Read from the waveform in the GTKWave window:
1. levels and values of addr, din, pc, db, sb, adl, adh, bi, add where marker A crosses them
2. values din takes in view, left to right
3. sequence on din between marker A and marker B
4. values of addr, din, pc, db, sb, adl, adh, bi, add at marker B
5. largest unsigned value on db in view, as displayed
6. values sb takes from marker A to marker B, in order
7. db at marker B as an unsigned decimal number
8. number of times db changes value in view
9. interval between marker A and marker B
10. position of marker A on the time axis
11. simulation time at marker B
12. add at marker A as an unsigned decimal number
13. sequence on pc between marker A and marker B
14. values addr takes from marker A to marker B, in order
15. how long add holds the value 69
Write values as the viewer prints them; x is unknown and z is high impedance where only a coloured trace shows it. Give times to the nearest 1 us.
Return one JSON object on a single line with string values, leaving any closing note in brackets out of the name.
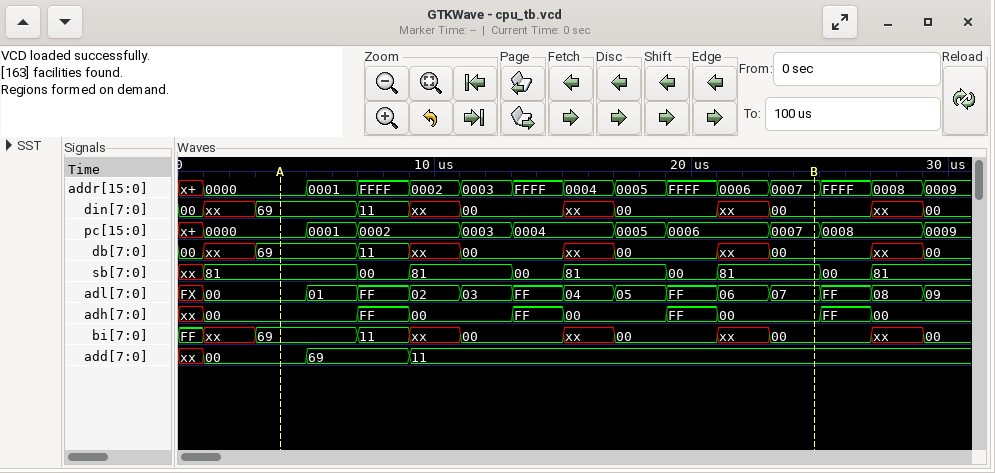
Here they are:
{"levels and values of addr, din, pc, db, sb, adl, adh, bi, add where marker A crosses them": "addr=0000, din=69, pc=0000, db=69, sb=81, adl=00, adh=00, bi=69, add=00", "values din takes in view, left to right": "00, xx, 69, 11, xx, 00, xx, 00, xx, 00, xx, 00", "sequence on din between marker A and marker B": "69, 11, xx, 00, xx, 00, xx, 00", "values of addr, din, pc, db, sb, adl, adh, bi, add at marker B": "addr=0007, din=00, pc=0007, db=00, sb=81, adl=07, adh=00, bi=00, add=11", "largest unsigned value on db in view, as displayed": "69", "values sb takes from marker A to marker B, in order": "81, 00, 81, 00, 81, 00, 81", "db at marker B as an unsigned decimal number": "0", "number of times db changes value in view": "11", "interval between marker A and marker B": "21 us", "position of marker A on the time axis": "4 us", "simulation time at marker B": "25 us", "add at marker A as an unsigned decimal number": "0", "sequence on pc between marker A and marker B": "0000, 0001, 0002, 0003, 0004, 0005, 0006, 0007", "values addr takes from marker A to marker B, in order": "0000, 0001, FFFF, 0002, 0003, FFFF, 0004, 0005, FFFF, 0006, 0007", "how long add holds the value 69": "4 us"}
